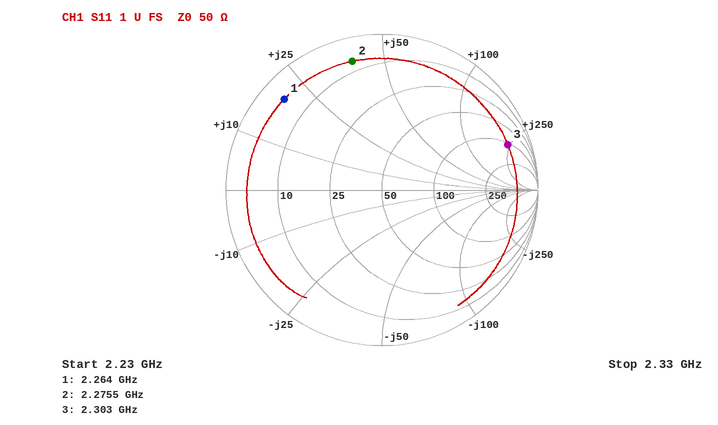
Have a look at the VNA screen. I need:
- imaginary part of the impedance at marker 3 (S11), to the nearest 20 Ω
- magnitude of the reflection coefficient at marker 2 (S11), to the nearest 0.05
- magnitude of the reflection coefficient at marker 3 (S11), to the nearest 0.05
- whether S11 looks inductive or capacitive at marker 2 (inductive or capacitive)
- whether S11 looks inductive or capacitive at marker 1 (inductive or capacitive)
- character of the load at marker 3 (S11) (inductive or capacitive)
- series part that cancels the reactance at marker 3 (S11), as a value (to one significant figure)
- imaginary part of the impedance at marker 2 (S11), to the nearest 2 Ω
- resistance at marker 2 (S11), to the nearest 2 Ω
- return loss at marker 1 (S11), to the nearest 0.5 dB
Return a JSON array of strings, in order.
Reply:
["+240 Ω", "0.85", "0.85", "inductive", "inductive", "inductive", "300 fF", "+40 Ω", "6 Ω", "1.5 dB"]
